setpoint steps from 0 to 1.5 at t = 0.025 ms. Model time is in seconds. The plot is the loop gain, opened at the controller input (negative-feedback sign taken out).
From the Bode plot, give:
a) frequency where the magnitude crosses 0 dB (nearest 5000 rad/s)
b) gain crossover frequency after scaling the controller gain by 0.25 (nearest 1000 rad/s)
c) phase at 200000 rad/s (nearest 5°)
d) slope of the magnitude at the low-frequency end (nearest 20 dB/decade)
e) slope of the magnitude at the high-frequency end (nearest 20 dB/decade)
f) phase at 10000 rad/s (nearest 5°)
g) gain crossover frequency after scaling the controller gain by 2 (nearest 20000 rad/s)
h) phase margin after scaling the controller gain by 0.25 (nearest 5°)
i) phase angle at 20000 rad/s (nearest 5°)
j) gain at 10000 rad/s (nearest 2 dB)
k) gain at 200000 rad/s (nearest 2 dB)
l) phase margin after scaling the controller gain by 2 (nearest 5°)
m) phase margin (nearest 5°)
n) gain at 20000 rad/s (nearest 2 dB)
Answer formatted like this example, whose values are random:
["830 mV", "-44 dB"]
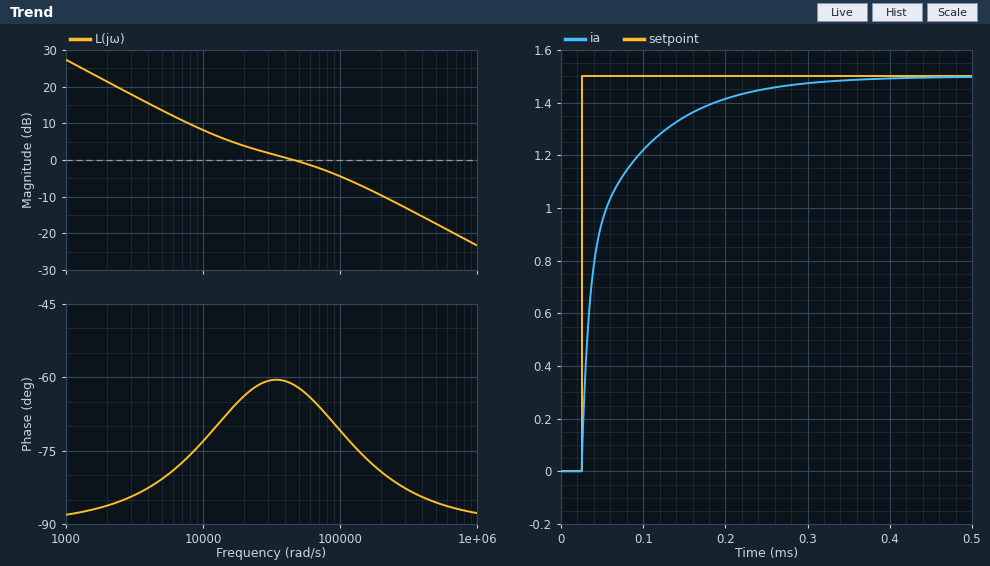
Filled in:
["45000 rad/s", "6000 rad/s", "-80°", "-20 dB/decade", "-20 dB/decade", "-75°", "120000 rad/s", "100°", "-65°", "8 dB", "-10 dB", "105°", "120°", "4 dB"]
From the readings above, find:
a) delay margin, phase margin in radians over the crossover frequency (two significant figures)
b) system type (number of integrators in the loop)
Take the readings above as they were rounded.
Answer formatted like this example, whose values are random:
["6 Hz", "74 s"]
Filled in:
["0.000047 s", "1"]
